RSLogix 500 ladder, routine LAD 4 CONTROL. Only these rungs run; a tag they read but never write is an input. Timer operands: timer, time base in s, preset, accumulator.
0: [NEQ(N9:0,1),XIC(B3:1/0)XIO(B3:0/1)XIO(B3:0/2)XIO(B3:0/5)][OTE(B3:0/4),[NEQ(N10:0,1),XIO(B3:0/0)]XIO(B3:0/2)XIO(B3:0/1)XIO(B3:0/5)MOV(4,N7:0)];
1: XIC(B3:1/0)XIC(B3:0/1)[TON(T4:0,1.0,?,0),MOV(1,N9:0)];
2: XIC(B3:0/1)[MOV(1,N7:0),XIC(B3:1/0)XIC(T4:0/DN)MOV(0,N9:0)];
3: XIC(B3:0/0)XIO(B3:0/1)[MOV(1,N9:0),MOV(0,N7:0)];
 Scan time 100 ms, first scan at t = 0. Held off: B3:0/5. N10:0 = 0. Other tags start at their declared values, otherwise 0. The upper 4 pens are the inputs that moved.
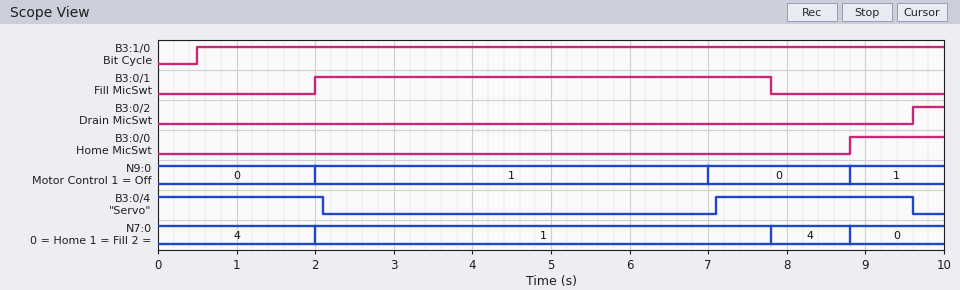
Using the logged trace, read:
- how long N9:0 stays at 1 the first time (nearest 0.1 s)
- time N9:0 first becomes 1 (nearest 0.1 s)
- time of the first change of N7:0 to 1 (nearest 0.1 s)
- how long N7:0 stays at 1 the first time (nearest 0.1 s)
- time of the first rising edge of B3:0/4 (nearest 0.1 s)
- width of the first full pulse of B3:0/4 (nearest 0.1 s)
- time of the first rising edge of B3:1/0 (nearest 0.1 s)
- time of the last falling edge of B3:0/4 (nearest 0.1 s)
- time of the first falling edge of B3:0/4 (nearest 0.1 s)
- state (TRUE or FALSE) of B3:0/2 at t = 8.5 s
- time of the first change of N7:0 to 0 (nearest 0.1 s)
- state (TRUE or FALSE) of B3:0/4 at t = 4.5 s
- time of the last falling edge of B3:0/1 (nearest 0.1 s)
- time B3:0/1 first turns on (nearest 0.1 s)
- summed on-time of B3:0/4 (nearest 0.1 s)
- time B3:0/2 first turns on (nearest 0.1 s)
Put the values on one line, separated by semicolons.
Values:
5.0 s; 2.0 s; 2.0 s; 5.8 s; 7.1 s; 2.5 s; 0.5 s; 9.6 s; 2.1 s; FALSE; 8.8 s; FALSE; 7.8 s; 2.0 s; 4.6 s; 9.6 s
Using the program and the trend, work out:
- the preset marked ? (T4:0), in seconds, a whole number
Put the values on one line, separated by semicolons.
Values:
5 s
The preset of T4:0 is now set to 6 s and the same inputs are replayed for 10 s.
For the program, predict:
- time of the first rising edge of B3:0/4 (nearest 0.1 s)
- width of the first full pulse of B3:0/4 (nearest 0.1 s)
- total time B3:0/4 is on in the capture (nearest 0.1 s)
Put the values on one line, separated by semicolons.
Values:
7.8 s; 1.8 s; 3.9 s
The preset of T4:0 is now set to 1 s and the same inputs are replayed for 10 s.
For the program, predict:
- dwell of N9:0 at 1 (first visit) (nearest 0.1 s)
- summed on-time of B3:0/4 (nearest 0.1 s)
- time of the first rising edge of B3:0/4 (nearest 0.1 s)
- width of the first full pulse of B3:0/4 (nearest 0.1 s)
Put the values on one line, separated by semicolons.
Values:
1.0 s; 8.6 s; 3.1 s; 6.5 s
